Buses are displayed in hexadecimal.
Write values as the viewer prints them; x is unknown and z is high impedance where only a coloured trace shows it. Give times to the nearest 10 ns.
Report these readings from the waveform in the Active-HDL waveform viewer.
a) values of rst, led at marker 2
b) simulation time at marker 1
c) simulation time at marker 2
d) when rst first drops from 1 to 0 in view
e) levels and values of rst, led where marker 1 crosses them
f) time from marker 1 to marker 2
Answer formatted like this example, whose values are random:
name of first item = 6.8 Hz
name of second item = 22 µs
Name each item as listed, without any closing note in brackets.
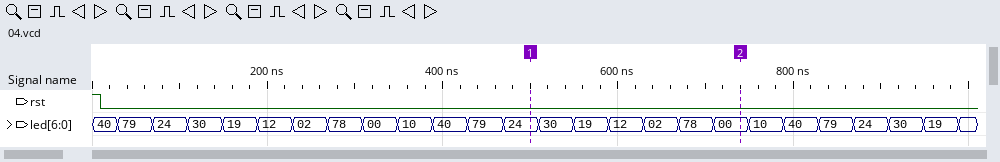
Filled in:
values of rst, led at marker 2 = rst=0, led=00
simulation time at marker 1 = 500 ns
simulation time at marker 2 = 740 ns
when rst first drops from 1 to 0 in view = 10 ns
levels and values of rst, led where marker 1 crosses them = rst=0, led=24
time from marker 1 to marker 2 = 240 ns
